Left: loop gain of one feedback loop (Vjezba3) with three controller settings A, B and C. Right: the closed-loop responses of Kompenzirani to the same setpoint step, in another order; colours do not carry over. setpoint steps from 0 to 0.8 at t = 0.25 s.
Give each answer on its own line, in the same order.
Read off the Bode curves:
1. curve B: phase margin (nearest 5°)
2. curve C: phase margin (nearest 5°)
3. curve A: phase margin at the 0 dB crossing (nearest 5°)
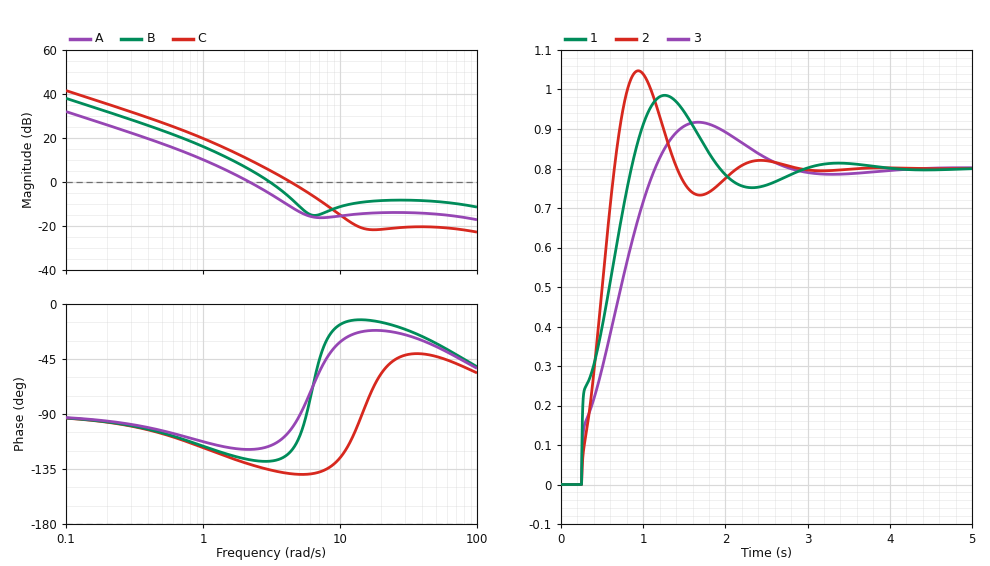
50°
40°
60°
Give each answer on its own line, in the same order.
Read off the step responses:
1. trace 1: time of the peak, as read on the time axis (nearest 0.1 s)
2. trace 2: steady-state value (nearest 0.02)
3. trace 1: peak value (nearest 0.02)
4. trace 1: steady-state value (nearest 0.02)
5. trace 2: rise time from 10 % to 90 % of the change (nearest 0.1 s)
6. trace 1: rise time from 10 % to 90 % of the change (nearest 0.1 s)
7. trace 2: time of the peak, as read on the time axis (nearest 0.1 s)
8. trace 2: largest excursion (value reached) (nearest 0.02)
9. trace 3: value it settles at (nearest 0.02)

1.3 s
0.80
0.98
0.80
0.3 s
0.5 s
0.9 s
1.04
0.80
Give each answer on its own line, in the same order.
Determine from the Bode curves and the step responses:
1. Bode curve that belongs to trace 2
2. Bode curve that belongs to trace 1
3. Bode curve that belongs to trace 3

C
B
A
